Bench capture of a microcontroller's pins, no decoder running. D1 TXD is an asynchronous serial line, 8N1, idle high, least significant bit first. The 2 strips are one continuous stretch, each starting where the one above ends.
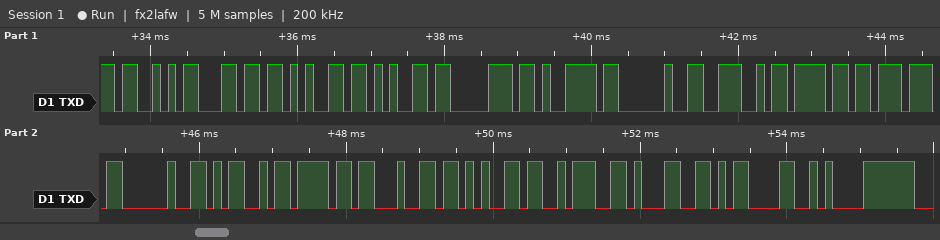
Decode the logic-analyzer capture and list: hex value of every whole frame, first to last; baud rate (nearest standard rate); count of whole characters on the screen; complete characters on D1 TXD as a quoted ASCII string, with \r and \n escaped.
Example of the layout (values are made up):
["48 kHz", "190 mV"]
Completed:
["0x53 0x6C 0x65 0x65 0x70 0x79 0x20 0x4E 0x6F 0x77 0x20 0x4D 0x6F 0x64 0x65 0x3A 0x31 0x0D 0x0A", "9600 baud", "19", "\"Sleepy Now Mode:1\\r\\n\""]
